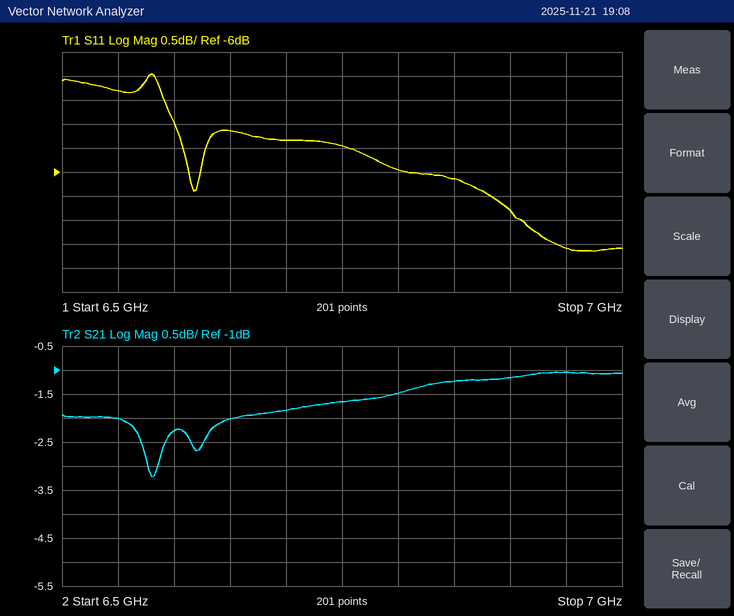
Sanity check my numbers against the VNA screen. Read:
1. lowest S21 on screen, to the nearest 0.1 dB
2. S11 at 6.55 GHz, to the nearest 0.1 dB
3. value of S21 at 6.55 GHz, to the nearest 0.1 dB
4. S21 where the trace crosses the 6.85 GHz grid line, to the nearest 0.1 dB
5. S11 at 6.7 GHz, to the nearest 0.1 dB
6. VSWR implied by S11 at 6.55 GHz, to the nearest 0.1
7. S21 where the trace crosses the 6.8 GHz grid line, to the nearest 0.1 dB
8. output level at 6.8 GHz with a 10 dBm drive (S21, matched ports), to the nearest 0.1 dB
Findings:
-3.2 dB
-4.3 dB
-2.0 dB
-1.2 dB
-5.3 dB
4.1
-1.5 dB
8.5 dBm
